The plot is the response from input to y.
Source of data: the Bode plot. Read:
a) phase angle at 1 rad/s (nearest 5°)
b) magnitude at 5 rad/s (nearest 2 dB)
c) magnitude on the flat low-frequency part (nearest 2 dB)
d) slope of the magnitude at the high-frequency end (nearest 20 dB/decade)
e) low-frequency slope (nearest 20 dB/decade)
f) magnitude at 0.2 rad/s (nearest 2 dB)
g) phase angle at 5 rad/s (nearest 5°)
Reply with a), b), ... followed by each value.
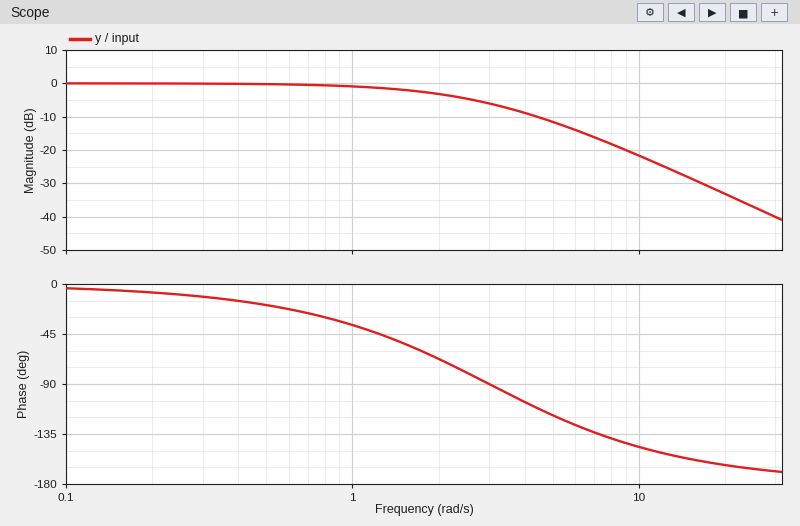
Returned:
a) -35°
b) -12 dB
c) 0 dB
d) -40 dB/decade
e) 0 dB/decade
f) 0 dB
g) -120°
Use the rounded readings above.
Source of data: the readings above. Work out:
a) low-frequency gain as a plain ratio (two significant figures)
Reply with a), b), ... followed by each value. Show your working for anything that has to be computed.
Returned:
a) 10^(0 / 20) = 1.0
